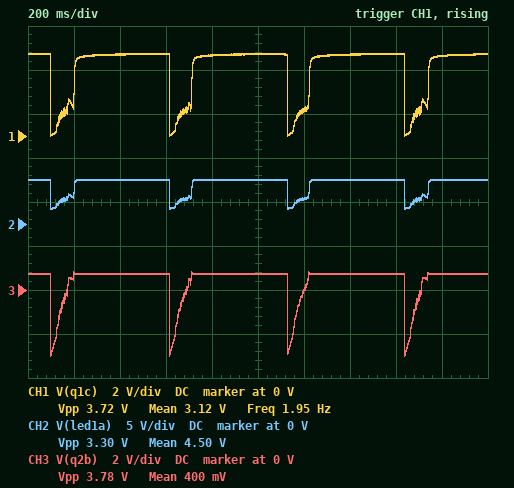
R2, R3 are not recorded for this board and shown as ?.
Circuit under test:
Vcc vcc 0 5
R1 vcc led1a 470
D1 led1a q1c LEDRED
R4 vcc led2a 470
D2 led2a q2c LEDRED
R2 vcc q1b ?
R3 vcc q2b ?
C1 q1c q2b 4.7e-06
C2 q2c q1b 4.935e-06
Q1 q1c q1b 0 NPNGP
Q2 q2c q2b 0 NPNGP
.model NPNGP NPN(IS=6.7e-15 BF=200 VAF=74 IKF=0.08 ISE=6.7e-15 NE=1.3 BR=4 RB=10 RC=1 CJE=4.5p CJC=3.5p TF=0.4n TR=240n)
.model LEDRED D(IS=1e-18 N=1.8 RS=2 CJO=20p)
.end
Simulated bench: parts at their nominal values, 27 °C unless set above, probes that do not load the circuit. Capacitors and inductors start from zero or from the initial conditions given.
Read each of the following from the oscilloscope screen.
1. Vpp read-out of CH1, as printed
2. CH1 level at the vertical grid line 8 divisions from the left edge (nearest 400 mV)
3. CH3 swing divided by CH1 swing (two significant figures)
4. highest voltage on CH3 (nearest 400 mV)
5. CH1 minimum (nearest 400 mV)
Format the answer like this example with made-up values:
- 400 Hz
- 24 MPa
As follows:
- 3.72 V
- 3.6 V
- 1.0
- 800 mV
- 0 V
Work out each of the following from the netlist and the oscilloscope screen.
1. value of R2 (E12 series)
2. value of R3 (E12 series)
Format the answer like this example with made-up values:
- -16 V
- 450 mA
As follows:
- 150 kΩ
- 56 kΩ
